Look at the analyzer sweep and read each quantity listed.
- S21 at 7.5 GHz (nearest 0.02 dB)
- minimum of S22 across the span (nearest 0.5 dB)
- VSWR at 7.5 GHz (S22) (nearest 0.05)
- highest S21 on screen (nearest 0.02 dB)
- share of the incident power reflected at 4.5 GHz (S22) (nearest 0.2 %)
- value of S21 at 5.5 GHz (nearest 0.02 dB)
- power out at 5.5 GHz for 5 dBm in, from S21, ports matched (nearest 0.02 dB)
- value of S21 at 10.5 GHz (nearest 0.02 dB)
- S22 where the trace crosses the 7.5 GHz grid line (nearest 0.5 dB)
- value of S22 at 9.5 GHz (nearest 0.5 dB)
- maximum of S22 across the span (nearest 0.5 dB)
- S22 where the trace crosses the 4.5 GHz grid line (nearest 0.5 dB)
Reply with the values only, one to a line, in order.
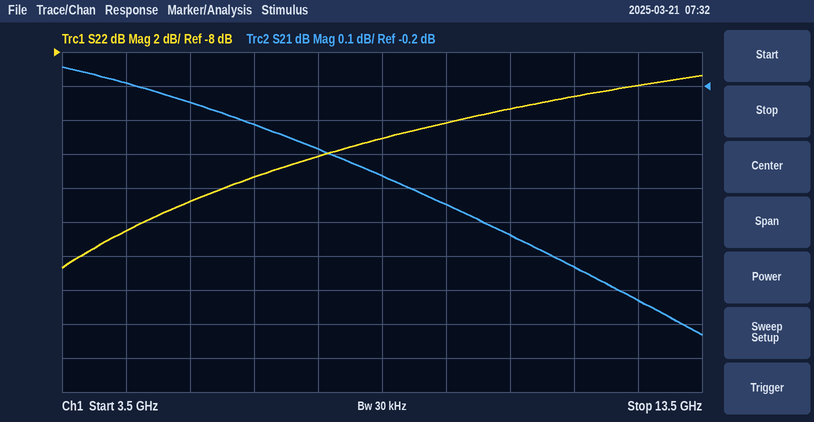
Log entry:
-0.38 dB
-20.5 dB
1.50
-0.14 dB
1.4 %
-0.24 dB
4.76 dBm
-0.64 dB
-14.0 dB
-12.0 dB
-9.5 dB
-18.5 dB
